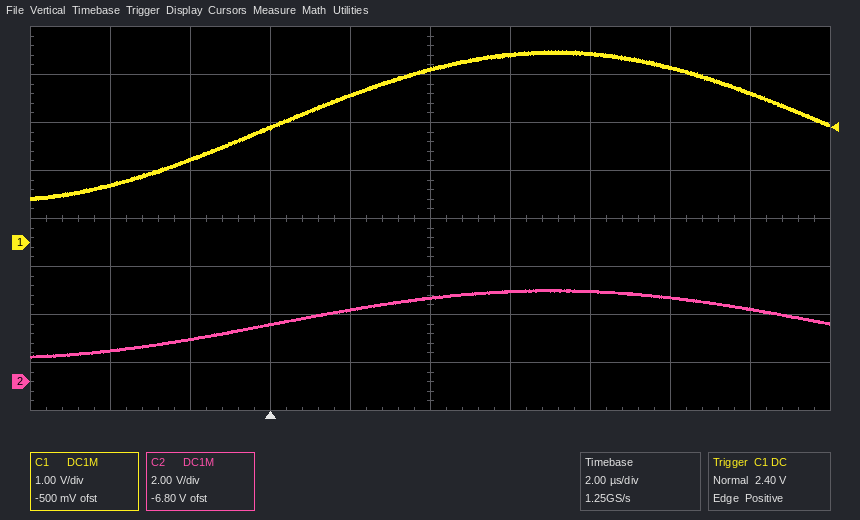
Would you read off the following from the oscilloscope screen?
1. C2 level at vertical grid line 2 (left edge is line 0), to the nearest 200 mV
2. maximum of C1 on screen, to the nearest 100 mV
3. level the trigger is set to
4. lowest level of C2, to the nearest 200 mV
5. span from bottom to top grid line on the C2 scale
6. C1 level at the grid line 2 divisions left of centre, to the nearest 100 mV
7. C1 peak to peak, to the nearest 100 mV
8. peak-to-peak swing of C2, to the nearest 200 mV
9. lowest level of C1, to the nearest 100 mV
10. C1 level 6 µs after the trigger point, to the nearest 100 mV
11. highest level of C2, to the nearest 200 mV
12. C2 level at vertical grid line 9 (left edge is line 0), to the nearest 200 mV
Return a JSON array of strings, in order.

["1.8 V", "4.0 V", "2.40 V", "1.0 V", "16 V", "2.4 V", "3.1 V", "2.8 V", "900 mV", "3.9 V", "3.8 V", "3.0 V"]
